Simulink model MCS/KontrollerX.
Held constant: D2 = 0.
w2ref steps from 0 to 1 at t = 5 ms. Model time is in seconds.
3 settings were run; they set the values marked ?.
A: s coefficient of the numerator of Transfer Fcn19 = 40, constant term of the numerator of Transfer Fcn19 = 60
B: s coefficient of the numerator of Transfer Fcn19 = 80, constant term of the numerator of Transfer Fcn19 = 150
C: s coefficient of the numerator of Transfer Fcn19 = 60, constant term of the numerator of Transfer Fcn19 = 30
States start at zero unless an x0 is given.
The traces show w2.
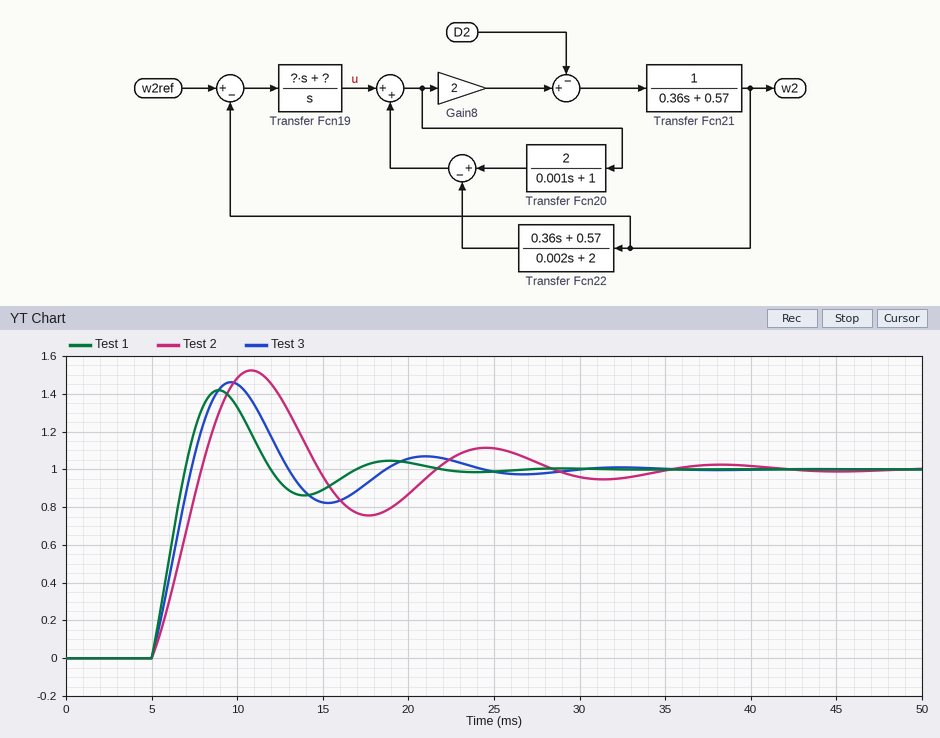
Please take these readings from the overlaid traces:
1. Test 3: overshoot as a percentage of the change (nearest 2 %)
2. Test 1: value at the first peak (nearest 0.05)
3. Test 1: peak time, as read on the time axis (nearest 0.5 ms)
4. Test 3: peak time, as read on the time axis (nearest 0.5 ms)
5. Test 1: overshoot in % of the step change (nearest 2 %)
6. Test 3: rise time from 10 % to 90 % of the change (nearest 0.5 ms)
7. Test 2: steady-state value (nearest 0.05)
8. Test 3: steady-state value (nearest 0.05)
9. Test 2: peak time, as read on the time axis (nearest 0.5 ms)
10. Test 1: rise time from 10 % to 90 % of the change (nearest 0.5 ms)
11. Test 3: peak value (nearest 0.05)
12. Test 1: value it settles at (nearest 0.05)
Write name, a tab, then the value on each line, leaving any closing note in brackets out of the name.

Test 3: overshoot as a percentage of the change	46 %
Test 1: value at the first peak	1.40
Test 1: peak time, as read on the time axis	9.0 ms
Test 3: peak time, as read on the time axis	9.5 ms
Test 1: overshoot in % of the step change	42 %
Test 3: rise time from 10 % to 90 % of the change	2.0 ms
Test 2: steady-state value	1.00
Test 3: steady-state value	1.00
Test 2: peak time, as read on the time axis	11.0 ms
Test 1: rise time from 10 % to 90 % of the change	1.5 ms
Test 3: peak value	1.45
Test 1: value it settles at	1.00
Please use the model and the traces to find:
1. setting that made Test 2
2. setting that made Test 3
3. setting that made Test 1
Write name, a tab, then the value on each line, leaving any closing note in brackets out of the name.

setting that made Test 2	A
setting that made Test 3	C
setting that made Test 1	B
